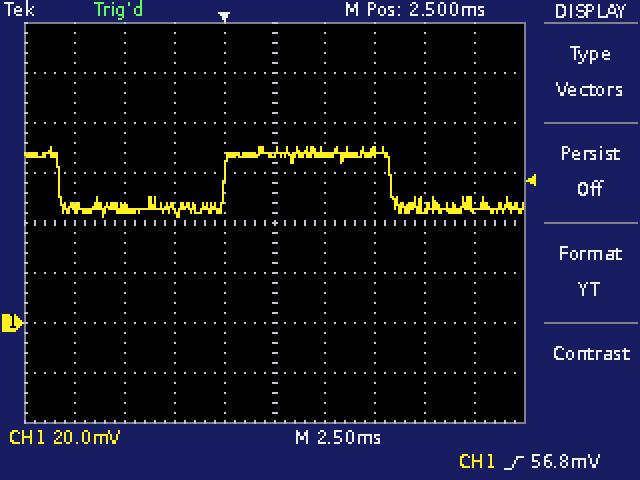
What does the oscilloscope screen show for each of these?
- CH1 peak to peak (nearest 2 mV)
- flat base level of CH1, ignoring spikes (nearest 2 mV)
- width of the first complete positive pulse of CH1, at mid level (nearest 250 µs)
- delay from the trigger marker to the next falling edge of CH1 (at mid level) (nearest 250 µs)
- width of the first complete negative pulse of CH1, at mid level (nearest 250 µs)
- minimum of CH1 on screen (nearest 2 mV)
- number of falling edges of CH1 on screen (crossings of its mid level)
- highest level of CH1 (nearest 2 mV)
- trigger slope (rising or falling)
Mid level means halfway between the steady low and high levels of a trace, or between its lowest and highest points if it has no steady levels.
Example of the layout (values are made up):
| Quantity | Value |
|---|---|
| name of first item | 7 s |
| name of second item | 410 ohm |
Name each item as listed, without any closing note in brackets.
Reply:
| Quantity | Value |
|---|---|
| CH1 peak to peak | 28 mV |
| flat base level of CH1, ignoring spikes | 46 mV |
| width of the first complete positive pulse of CH1, at mid level | 8.25 ms |
| delay from the trigger marker to the next falling edge of CH1 (at mid level) | 8.25 ms |
| width of the first complete negative pulse of CH1, at mid level | 8.25 ms |
| minimum of CH1 on screen | 42 mV |
| number of falling edges of CH1 on screen | 2 |
| highest level of CH1 | 70 mV |
| trigger slope | rising |
